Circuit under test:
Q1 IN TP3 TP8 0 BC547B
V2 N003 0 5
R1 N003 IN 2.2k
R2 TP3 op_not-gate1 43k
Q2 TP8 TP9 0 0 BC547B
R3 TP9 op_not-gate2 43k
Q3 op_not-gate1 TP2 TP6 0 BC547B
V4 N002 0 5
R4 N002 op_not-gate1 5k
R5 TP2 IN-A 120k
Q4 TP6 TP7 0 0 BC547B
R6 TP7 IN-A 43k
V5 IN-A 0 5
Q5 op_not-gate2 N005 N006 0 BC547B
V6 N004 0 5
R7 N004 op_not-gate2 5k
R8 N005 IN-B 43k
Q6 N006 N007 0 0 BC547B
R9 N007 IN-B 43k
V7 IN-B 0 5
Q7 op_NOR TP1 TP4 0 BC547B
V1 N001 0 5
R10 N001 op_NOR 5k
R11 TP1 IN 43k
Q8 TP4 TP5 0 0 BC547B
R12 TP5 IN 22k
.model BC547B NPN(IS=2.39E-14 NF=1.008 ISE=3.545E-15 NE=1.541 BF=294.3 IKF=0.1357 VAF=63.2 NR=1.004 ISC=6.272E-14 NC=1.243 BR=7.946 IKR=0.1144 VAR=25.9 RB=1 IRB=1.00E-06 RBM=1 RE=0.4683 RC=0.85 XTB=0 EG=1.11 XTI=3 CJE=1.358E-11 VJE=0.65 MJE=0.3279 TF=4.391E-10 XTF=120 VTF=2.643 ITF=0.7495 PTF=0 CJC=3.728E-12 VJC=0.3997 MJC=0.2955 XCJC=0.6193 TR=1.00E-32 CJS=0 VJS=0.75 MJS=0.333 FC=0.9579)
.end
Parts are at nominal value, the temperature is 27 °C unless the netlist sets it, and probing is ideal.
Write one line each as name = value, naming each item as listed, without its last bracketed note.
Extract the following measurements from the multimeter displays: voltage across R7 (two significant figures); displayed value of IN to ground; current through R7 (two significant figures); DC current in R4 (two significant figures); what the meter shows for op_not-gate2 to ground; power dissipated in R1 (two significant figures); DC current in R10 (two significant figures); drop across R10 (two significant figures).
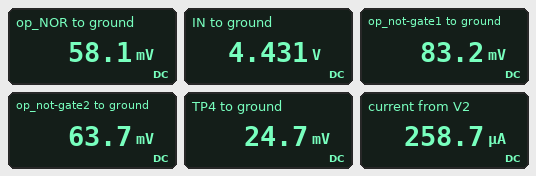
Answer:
voltage across R7 = 4.9 V
displayed value of IN to ground = 4.431 V
current through R7 = 990 µA
DC current in R4 = 980 µA
what the meter shows for op_not-gate2 to ground = 63.7 mV
power dissipated in R1 = 150 µW
DC current in R10 = 990 µA
drop across R10 = 4.9 V
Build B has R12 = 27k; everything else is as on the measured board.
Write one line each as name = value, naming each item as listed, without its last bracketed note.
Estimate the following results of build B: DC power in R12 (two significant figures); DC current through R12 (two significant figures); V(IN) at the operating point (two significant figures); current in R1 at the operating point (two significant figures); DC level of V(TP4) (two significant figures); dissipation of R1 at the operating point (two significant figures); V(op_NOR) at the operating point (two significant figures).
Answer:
DC power in R12 = 540 µW
DC current through R12 = 140 µA
V(IN) at the operating point = 4.5 V
current in R1 at the operating point = 230 µA
DC level of V(TP4) = 27 mV
dissipation of R1 at the operating point = 120 µW
V(op_NOR) at the operating point = 60 mV
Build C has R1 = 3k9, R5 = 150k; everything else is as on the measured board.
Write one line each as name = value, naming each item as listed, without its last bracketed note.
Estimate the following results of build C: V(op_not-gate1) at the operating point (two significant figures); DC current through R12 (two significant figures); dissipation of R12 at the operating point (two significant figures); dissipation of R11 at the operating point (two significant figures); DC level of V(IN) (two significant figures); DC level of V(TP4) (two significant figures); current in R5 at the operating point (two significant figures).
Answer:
V(op_not-gate1) at the operating point = 89 mV
DC current through R12 = 160 µA
dissipation of R12 at the operating point = 530 µW
dissipation of R11 at the operating point = 270 µW
DC level of V(IN) = 4.1 V
DC level of V(TP4) = 26 mV
current in R5 at the operating point = 29 µA
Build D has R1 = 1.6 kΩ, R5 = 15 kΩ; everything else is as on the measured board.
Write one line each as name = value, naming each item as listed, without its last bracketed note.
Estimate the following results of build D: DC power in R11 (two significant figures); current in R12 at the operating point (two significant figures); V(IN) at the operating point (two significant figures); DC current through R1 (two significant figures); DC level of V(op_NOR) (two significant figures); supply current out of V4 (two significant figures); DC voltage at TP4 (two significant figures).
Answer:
DC power in R11 = 350 µW
current in R12 at the operating point = 180 µA
V(IN) at the operating point = 4.6 V
DC current through R1 = 270 µA
DC level of V(op_NOR) = 57 mV
supply current out of V4 = 990 µA
DC voltage at TP4 = 24 mV
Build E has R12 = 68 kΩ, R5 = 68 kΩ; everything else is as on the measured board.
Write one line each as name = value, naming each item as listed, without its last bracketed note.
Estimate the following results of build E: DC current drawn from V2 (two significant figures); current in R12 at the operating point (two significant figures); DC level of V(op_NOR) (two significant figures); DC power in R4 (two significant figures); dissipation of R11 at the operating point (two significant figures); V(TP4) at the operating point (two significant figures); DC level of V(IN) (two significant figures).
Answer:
DC current drawn from V2 = 150 µA
current in R12 at the operating point = 59 µA
DC level of V(op_NOR) = 75 mV
DC power in R4 = 4.9 mW
dissipation of R11 at the operating point = 370 µW
V(TP4) at the operating point = 43 mV
DC level of V(IN) = 4.7 V
